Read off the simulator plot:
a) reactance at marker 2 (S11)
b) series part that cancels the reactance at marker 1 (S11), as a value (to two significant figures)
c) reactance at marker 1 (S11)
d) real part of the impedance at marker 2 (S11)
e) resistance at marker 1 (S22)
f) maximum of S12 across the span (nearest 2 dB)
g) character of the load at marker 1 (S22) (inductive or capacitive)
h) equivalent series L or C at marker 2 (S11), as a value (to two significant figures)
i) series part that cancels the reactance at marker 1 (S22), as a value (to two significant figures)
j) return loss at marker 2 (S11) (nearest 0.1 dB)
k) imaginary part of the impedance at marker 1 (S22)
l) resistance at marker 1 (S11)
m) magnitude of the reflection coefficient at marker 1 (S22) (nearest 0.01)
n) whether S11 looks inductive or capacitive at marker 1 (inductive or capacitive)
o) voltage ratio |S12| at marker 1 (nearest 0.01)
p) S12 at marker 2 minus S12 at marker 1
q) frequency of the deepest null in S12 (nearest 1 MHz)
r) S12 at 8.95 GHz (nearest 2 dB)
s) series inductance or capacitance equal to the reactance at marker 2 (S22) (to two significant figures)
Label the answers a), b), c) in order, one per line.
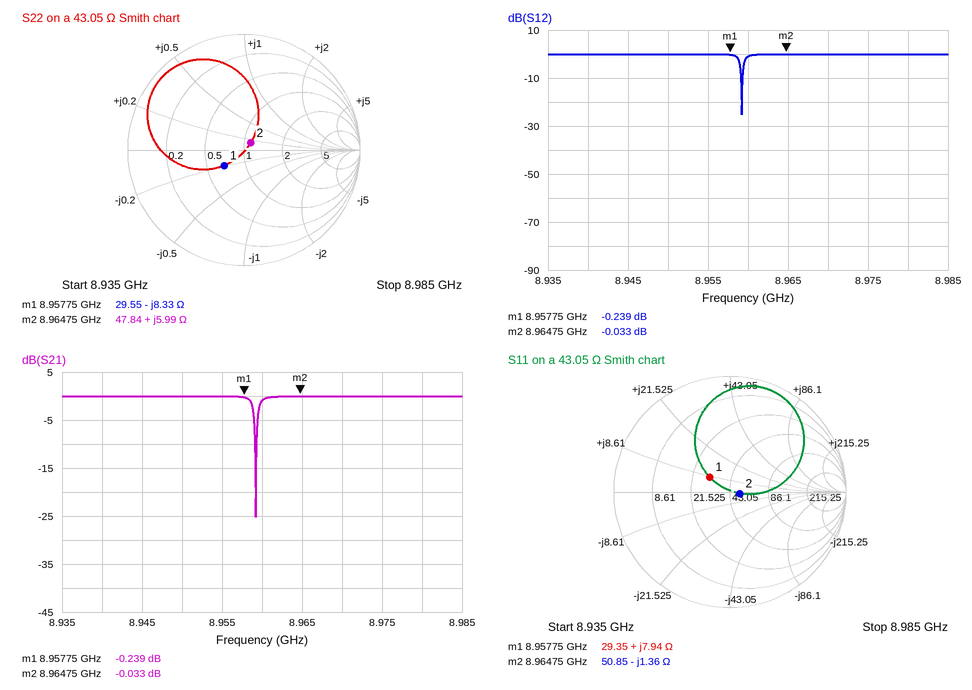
a) -1.36 Ω
b) 2.2 pF
c) +7.94 Ω
d) 50.85 Ω
e) 29.55 Ω
f) 0 dB
g) capacitive
h) 13 pF
i) 150 pH
j) 21.5 dB
k) -8.33 Ω
l) 29.35 Ω
m) 0.22
n) inductive
o) 0.97
p) 0.206 dB
q) 8.959 GHz
r) 0 dB
s) 110 pH
